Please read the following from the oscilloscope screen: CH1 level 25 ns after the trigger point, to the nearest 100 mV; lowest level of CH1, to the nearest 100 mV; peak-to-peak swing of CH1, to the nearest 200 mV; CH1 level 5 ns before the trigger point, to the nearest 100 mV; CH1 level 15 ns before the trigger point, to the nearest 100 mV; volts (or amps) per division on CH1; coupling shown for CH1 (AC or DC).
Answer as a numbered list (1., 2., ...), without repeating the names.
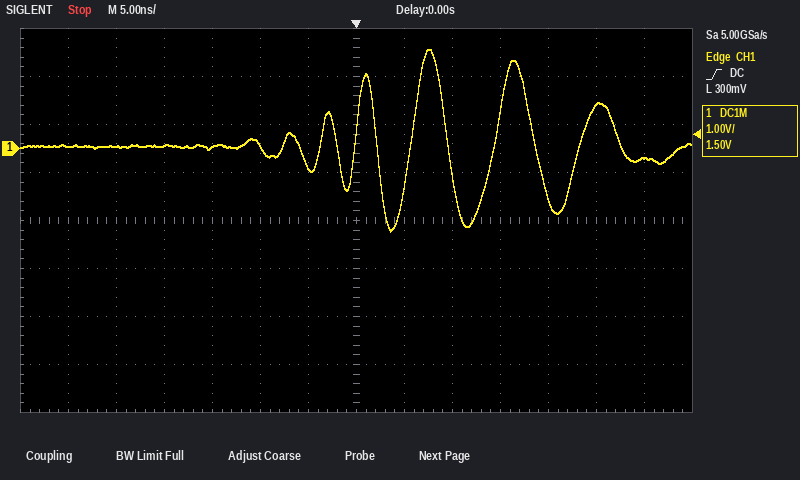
1. 900 mV
2. -1.7 V
3. 3.8 V
4. -400 mV
5. 0.0 V
6. 1 V
7. DC
